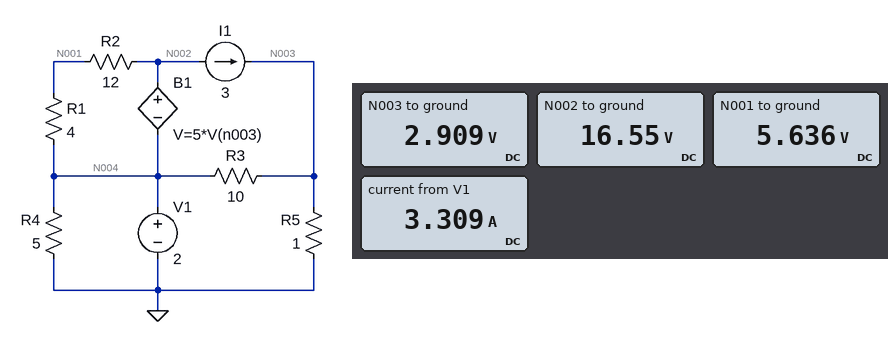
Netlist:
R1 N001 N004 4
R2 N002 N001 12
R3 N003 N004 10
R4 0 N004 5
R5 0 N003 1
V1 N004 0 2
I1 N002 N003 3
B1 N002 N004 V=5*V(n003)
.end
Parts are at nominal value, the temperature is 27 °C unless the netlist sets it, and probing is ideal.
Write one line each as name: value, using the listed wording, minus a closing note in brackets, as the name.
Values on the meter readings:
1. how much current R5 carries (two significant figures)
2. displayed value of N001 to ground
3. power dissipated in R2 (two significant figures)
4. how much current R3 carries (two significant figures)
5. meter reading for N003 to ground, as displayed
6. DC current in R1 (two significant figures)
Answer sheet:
how much current R5 carries: 2.9 A
displayed value of N001 to ground: 5.636 V
power dissipated in R2: 9.9 W
how much current R3 carries: 91 mA
meter reading for N003 to ground, as displayed: 2.909 V
DC current in R1: 910 mA
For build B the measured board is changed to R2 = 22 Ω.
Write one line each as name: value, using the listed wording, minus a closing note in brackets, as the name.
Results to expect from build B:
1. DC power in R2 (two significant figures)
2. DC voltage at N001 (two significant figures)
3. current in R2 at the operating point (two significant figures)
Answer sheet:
DC power in R2: 6.9 W
DC voltage at N001: 4.2 V
current in R2 at the operating point: 560 mA
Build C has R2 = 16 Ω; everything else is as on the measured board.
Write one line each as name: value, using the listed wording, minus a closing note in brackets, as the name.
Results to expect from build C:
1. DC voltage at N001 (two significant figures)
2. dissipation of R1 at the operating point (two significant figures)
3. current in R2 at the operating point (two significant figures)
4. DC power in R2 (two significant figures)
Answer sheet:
DC voltage at N001: 4.9 V
dissipation of R1 at the operating point: 2.1 W
current in R2 at the operating point: 730 mA
DC power in R2: 8.5 W
